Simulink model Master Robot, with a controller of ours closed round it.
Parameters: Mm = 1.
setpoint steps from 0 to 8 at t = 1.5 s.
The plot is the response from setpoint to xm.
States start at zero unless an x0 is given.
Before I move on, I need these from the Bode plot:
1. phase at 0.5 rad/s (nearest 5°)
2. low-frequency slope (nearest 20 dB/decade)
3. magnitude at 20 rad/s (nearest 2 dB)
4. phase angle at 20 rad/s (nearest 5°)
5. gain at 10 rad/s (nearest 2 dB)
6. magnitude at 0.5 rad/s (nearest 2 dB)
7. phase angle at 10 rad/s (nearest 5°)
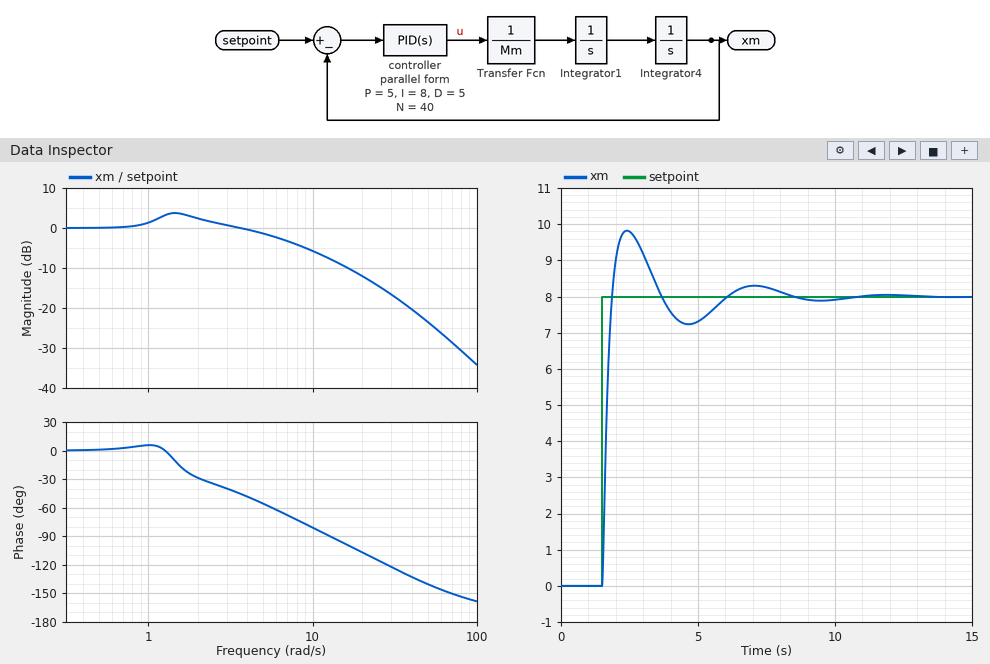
0°
0 dB/decade
-12 dB
-105°
-6 dB
0 dB
-80°
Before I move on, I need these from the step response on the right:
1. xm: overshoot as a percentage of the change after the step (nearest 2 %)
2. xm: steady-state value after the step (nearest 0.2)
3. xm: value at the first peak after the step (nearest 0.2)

22 %
8.0
9.8
